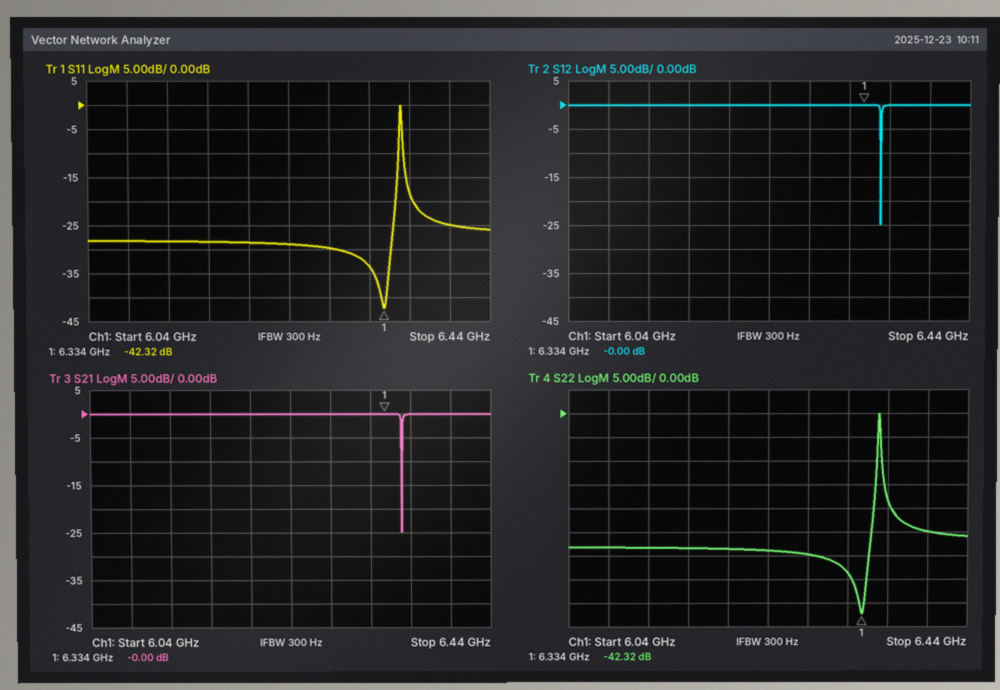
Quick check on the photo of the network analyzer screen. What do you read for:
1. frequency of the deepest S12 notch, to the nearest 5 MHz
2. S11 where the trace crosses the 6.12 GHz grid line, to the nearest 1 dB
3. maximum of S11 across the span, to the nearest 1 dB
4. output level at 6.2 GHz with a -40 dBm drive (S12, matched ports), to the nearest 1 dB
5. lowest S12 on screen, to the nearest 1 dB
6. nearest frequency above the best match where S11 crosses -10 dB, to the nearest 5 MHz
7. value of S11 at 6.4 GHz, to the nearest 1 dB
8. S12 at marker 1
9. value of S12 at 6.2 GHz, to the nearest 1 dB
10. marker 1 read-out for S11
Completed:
6.350 GHz
-28 dB
0 dB
-40 dBm
-25 dB
6.350 GHz
-25 dB
-0.00 dB
0 dB
-42.32 dB
